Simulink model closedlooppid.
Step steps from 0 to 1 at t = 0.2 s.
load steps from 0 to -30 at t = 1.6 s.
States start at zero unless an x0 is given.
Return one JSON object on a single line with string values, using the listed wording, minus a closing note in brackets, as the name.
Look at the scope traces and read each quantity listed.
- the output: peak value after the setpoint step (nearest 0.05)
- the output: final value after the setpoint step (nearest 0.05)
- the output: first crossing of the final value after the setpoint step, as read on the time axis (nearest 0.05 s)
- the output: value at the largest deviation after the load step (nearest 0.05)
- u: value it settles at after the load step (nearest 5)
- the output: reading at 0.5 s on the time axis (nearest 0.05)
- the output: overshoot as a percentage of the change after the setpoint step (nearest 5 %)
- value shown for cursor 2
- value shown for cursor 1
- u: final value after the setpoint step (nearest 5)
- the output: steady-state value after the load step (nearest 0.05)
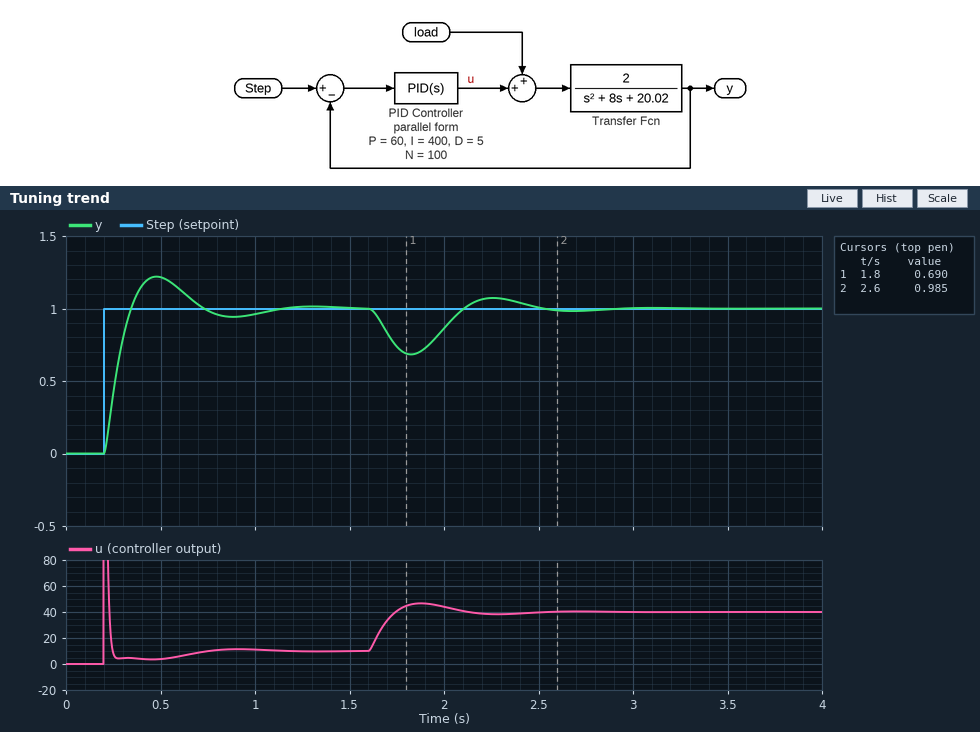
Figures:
{"the output: peak value after the setpoint step": "1.20", "the output: final value after the setpoint step": "1.00", "the output: first crossing of the final value after the setpoint step, as read on the time axis": "0.35 s", "the output: value at the largest deviation after the load step": "0.70", "u: value it settles at after the load step": "40", "the output: reading at 0.5 s on the time axis": "1.20", "the output: overshoot as a percentage of the change after the setpoint step": "20 %", "value shown for cursor 2": "0.985", "value shown for cursor 1": "0.690", "u: final value after the setpoint step": "10", "the output: steady-state value after the load step": "1.00"}
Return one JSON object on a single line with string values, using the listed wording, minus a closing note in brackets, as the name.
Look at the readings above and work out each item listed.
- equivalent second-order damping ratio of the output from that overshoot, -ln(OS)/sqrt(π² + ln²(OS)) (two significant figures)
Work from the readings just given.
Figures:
{"equivalent second-order damping ratio of the output from that overshoot, -ln(OS)/sqrt(π² + ln²(OS))": "0.46"}
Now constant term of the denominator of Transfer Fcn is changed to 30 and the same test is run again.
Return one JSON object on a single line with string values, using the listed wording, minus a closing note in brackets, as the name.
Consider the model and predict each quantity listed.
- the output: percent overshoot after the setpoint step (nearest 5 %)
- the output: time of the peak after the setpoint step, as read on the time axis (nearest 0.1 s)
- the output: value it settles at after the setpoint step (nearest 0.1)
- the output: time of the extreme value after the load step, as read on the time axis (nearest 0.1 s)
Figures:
{"the output: percent overshoot after the setpoint step": "15 %", "the output: time of the peak after the setpoint step, as read on the time axis": "0.5 s", "the output: value it settles at after the setpoint step": "1.0", "the output: time of the extreme value after the load step, as read on the time axis": "1.8 s"}
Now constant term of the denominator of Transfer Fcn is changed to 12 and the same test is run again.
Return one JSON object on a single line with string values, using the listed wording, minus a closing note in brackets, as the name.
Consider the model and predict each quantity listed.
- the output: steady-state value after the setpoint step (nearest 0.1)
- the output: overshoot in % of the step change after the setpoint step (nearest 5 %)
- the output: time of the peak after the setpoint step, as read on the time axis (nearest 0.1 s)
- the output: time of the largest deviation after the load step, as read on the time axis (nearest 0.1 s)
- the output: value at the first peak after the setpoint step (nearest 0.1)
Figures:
{"the output: steady-state value after the setpoint step": "1.0", "the output: overshoot in % of the step change after the setpoint step": "25 %", "the output: time of the peak after the setpoint step, as read on the time axis": "0.5 s", "the output: time of the largest deviation after the load step, as read on the time axis": "1.8 s", "the output: value at the first peak after the setpoint step": "1.3"}
